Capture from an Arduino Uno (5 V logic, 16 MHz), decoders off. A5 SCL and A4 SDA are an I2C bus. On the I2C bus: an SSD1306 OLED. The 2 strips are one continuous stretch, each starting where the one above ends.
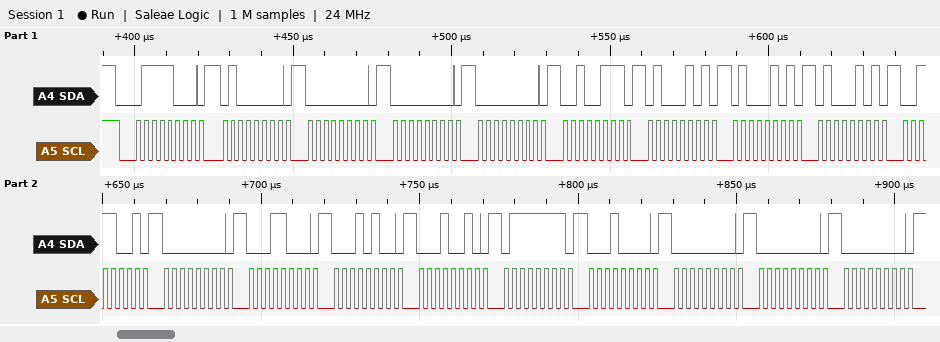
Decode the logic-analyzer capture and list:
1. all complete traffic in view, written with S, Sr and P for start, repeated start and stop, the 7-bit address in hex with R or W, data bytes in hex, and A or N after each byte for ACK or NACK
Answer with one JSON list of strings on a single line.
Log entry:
["S 3CW A 40 A 00 A 00 A 00 A 27 A 45 A 45 A 45 A 39 A 00 A 18 A 14 A 12 A 7F A 10 A 00 A 00 A 00 A"]
